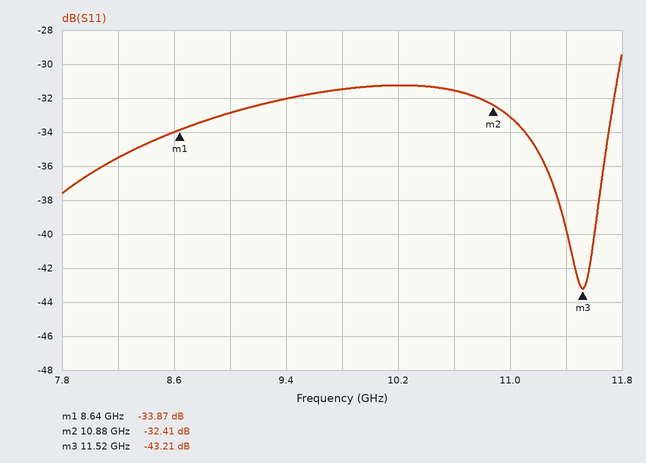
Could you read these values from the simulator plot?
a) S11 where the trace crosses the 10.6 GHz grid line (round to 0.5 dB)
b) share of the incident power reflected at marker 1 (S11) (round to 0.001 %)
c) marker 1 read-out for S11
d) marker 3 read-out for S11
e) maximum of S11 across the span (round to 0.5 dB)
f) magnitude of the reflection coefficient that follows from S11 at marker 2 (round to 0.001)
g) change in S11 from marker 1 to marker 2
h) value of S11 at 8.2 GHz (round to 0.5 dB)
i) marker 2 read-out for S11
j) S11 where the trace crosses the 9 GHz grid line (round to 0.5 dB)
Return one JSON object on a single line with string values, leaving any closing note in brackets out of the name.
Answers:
{"S11 where the trace crosses the 10.6 GHz grid line": "-31.5 dB", "share of the incident power reflected at marker 1 (S11)": "0.041 %", "marker 1 read-out for S11": "-33.87 dB", "marker 3 read-out for S11": "-43.21 dB", "maximum of S11 across the span": "-29.5 dB", "magnitude of the reflection coefficient that follows from S11 at marker 2": "0.024", "change in S11 from marker 1 to marker 2": "1.46 dB", "value of S11 at 8.2 GHz": "-35.5 dB", "marker 2 read-out for S11": "-32.41 dB", "S11 where the trace crosses the 9 GHz grid line": "-33.0 dB"}
